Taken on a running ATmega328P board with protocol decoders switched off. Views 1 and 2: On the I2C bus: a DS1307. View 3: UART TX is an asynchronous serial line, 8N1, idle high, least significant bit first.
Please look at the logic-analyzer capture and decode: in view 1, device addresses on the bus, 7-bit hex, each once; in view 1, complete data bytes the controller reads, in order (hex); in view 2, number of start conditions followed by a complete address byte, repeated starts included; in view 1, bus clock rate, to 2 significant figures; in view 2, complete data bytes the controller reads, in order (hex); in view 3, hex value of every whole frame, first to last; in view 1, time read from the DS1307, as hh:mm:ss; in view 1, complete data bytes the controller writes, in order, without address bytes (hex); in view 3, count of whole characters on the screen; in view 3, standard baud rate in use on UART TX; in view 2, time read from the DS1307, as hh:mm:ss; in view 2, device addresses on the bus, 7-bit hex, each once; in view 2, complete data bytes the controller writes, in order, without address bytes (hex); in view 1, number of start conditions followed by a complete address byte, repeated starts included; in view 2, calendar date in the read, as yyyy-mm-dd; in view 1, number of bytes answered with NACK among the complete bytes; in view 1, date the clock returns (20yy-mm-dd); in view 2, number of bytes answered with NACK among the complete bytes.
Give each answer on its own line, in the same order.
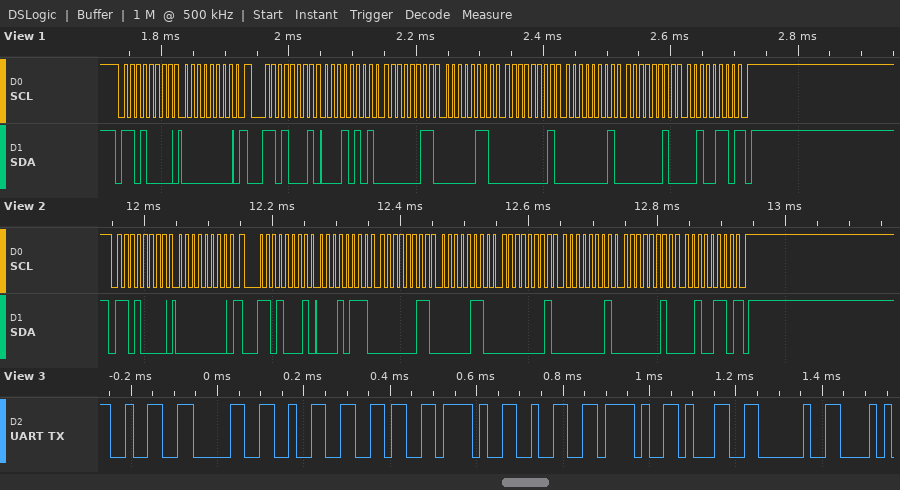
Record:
0x68
15 03 06 01 01 02 26
2
100 kHz
17 03 06 01 01 02 26
32 30 32 36 2F 32 2F 31 20
06:03:15
00
9
57600 baud
06:03:17
0x68
00
2
2026-02-01
1
2026-02-01
1
